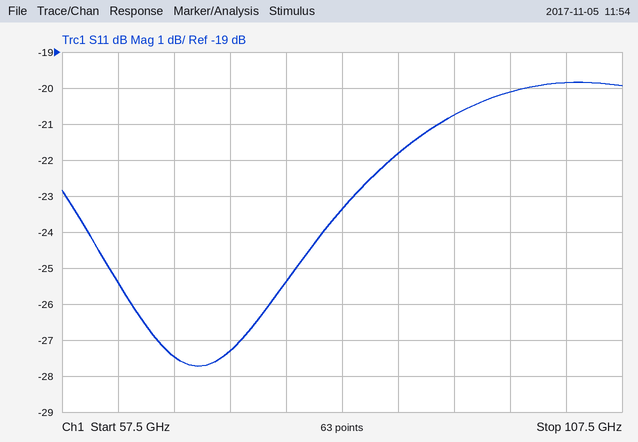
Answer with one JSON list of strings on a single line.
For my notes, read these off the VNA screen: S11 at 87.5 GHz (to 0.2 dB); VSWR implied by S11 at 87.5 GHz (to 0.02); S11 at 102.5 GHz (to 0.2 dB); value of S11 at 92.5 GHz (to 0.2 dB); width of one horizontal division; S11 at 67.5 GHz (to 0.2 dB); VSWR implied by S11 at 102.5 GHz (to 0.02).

["-21.8 dB", "1.18", "-19.8 dB", "-20.8 dB", "5 GHz", "-27.4 dB", "1.22"]
